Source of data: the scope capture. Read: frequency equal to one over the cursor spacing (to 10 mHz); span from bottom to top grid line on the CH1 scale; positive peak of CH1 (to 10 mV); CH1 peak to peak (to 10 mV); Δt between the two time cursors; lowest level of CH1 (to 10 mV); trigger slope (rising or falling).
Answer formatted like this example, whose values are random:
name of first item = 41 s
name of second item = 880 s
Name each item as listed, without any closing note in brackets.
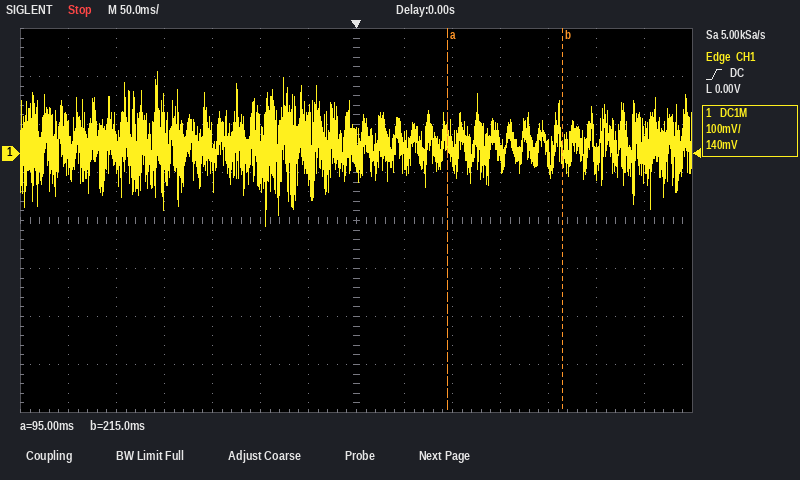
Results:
frequency equal to one over the cursor spacing = 8.33 Hz
span from bottom to top grid line on the CH1 scale = 800 mV
positive peak of CH1 = 170 mV
CH1 peak to peak = 320 mV
Δt between the two time cursors = 120 ms
lowest level of CH1 = -150 mV
trigger slope = rising
